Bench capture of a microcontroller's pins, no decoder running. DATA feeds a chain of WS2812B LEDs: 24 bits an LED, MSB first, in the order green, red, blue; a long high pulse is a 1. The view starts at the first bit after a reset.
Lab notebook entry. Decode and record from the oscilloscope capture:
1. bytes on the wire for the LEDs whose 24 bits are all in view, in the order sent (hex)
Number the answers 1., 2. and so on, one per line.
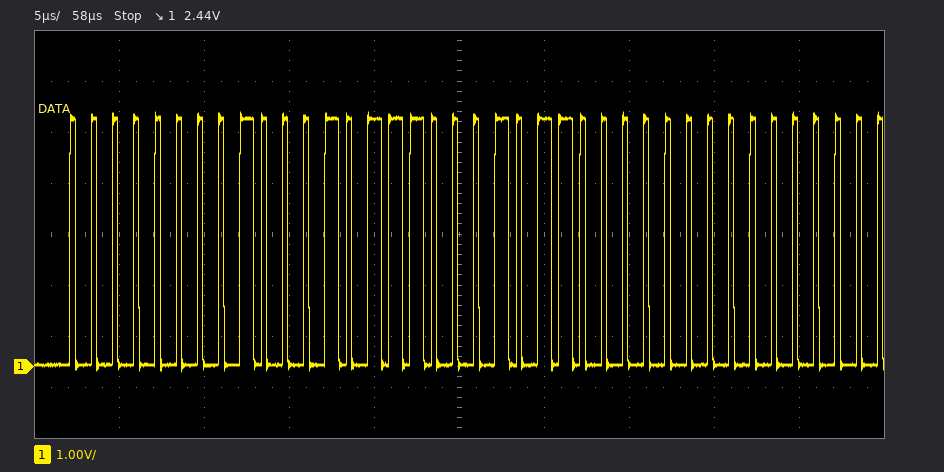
1. 00 8B 8B
